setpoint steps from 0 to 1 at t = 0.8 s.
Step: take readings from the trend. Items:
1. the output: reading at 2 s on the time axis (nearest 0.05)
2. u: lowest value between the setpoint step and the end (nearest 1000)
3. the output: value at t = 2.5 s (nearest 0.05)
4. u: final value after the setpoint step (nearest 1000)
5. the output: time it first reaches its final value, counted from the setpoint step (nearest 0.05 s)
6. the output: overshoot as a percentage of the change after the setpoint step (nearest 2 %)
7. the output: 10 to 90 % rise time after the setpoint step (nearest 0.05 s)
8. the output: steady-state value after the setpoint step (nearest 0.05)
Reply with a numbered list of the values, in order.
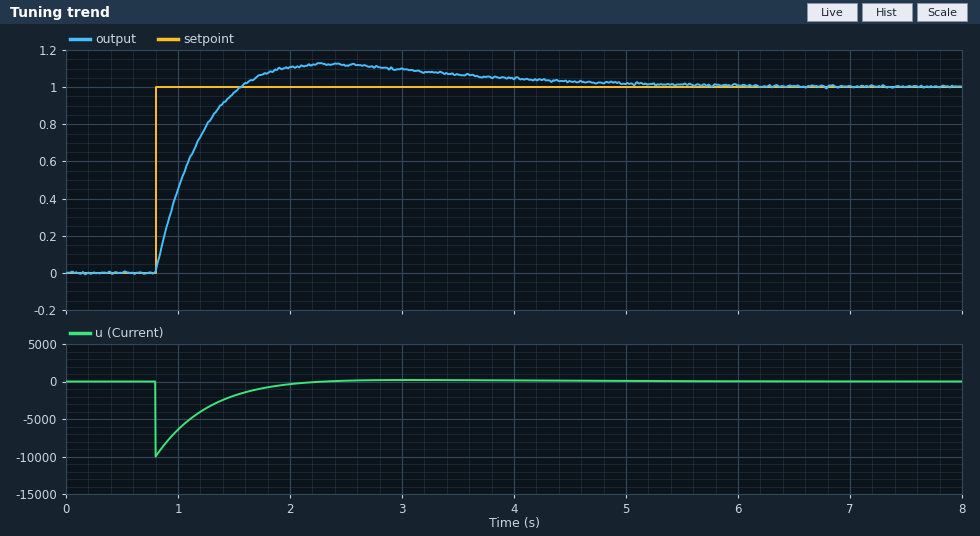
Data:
1. 1.10
2. -10000
3. 1.10
4. 0
5. 0.75 s
6. 12 %
7. 0.55 s
8. 1.00
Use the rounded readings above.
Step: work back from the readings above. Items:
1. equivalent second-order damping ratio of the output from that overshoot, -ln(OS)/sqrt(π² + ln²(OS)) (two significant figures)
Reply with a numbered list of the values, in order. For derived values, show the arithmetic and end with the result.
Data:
1. ln(0.12) = -2.120; 2.120 / sqrt(9.870 + 4.496) = 0.56
